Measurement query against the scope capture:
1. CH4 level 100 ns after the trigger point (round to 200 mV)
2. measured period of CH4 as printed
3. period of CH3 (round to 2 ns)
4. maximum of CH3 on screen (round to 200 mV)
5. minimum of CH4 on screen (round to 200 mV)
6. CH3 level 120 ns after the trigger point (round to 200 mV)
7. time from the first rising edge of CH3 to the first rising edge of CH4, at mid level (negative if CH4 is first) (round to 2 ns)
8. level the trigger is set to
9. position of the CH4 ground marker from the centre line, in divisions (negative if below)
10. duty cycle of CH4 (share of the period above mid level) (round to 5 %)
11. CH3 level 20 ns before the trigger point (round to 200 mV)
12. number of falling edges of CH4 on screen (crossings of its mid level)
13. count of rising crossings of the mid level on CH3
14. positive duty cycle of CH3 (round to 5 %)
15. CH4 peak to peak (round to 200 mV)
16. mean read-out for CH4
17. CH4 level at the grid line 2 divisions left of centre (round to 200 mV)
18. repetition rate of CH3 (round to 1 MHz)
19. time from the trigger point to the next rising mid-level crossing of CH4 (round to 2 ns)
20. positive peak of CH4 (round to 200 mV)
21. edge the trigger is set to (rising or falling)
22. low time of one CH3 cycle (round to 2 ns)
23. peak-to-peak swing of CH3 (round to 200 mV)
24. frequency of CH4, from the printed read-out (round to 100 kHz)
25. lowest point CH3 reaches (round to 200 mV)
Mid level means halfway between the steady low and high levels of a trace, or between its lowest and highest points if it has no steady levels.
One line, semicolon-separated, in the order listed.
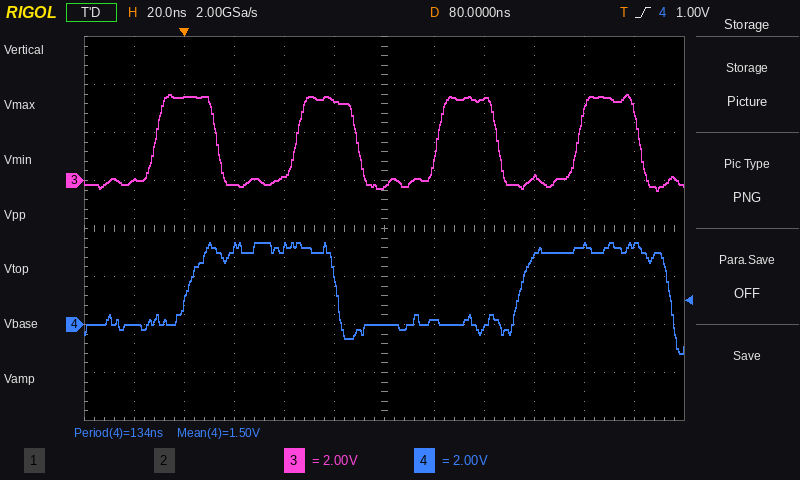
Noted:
200 mV; 134 ns; 56 ns; 3.6 V; -1.2 V; 3.4 V; +12 ns; 1.00 V; -2.0 div; 45 %; 0.0 V; 2; 4; 45 %; 4.6 V; 1.50 V; 3.2 V; 18 MHz; 134 ns; 3.4 V; rising; 32 ns; 4.0 V; 7.5 MHz; -400 mV
